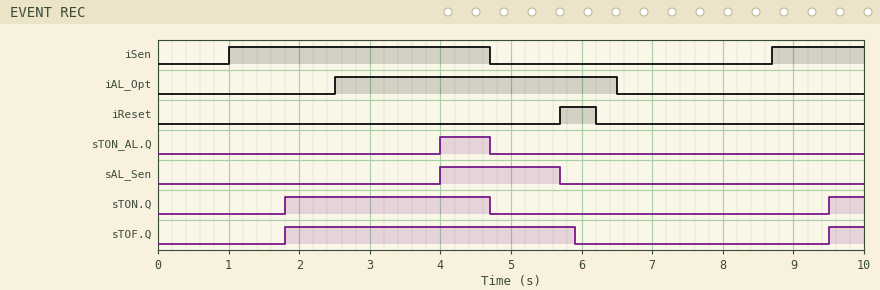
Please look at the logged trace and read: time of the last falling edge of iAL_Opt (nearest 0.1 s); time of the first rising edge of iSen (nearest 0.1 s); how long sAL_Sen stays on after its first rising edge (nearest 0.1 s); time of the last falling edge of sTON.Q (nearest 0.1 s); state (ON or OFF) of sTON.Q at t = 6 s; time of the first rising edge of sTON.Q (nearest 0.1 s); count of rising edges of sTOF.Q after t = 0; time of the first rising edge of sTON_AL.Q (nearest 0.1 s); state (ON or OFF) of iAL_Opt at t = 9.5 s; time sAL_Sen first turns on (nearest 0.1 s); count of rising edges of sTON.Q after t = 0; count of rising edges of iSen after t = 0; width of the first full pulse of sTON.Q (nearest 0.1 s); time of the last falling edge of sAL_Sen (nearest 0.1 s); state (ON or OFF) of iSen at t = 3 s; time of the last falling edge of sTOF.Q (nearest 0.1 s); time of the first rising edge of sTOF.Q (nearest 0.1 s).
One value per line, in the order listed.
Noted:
6.5 s
1.0 s
1.7 s
4.7 s
OFF
1.8 s
2
4.0 s
OFF
4.0 s
2
2
2.9 s
5.7 s
ON
5.9 s
1.8 s
